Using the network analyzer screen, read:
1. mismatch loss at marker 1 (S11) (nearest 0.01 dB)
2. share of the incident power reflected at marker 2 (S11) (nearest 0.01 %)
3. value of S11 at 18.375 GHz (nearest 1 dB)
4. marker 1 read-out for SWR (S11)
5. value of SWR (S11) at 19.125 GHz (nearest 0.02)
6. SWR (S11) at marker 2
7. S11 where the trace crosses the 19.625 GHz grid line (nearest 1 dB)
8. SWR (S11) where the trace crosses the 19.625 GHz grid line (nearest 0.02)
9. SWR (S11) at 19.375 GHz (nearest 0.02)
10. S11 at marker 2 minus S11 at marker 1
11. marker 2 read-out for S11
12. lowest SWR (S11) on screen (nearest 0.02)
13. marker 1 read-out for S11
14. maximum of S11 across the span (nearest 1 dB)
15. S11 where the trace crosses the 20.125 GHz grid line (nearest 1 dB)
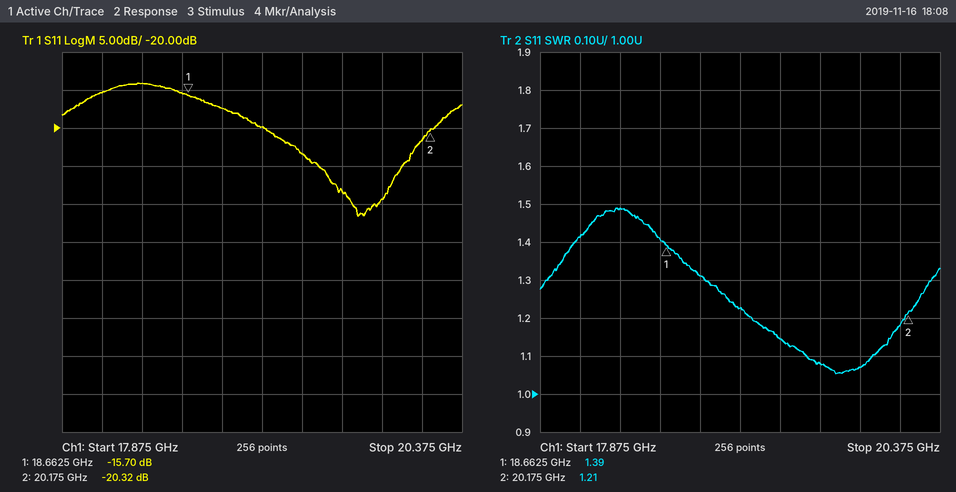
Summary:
0.12 dB
0.93 %
-14 dB
1.39
1.22
1.21
-28 dB
1.08
1.14
-4.62 dB
-20.32 dB
1.06
-15.70 dB
-14 dB
-22 dB
